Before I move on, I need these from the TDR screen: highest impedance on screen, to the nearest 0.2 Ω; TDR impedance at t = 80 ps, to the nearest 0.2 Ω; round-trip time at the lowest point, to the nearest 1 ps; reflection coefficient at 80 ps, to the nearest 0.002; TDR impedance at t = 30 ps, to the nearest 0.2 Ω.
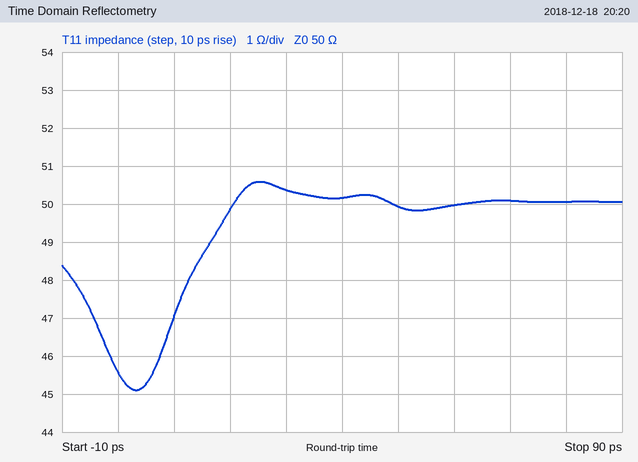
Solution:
50.6 Ω
50.0 Ω
3 ps
0.000
50.4 Ω
